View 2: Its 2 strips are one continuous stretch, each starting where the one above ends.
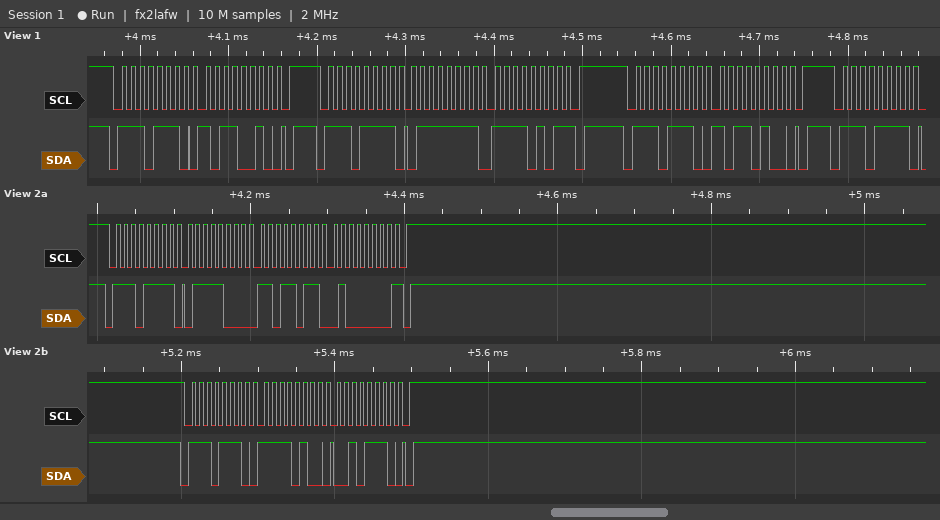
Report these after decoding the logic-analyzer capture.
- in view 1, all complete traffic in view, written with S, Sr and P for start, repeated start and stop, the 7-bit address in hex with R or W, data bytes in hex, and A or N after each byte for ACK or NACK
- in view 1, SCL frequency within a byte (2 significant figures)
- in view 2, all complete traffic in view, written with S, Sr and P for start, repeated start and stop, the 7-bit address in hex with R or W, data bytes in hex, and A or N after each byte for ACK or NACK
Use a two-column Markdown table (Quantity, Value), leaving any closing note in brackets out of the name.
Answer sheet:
| Quantity | Value |
|---|---|
| in view 1, all complete traffic in view, written with S, Sr and P for start, repeated start and stop, the 7-bit address in hex with R or W, data bytes in hex, and A or N after each byte for ACK or NACK | S 77W A B2 A P S 77R A 7F A F5 N P S 77W A B4 A P S 77R A |
| in view 1, SCL frequency within a byte | 100 kHz |
| in view 2, all complete traffic in view, written with S, Sr and P for start, repeated start and stop, the 7-bit address in hex with R or W, data bytes in hex, and A or N after each byte for ACK or NACK | S 77R A 78 A DB A 40 N P S 77W A F4 A 2E A P |
